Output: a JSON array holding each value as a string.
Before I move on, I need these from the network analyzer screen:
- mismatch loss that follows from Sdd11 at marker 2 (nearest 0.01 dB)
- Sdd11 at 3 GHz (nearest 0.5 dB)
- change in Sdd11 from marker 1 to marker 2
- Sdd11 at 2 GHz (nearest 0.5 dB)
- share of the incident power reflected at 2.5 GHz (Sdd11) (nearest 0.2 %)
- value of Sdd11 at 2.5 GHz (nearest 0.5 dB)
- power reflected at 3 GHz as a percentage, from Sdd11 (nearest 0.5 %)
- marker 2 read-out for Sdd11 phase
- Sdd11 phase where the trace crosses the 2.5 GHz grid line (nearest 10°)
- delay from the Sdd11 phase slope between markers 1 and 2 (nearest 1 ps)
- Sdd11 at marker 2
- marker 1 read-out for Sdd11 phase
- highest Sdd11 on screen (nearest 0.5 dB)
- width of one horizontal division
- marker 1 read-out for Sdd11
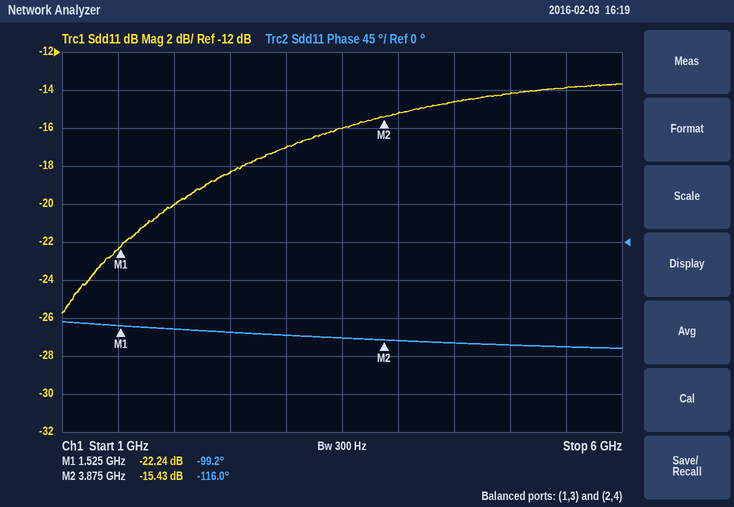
["0.13 dB", "-17.0 dB", "6.81 dB", "-20.0 dB", "1.4 %", "-18.5 dB", "2.0 %", "-116.0°", "-110°", "20 ps", "-15.43 dB", "-99.2°", "-13.5 dB", "500 MHz", "-22.24 dB"]
